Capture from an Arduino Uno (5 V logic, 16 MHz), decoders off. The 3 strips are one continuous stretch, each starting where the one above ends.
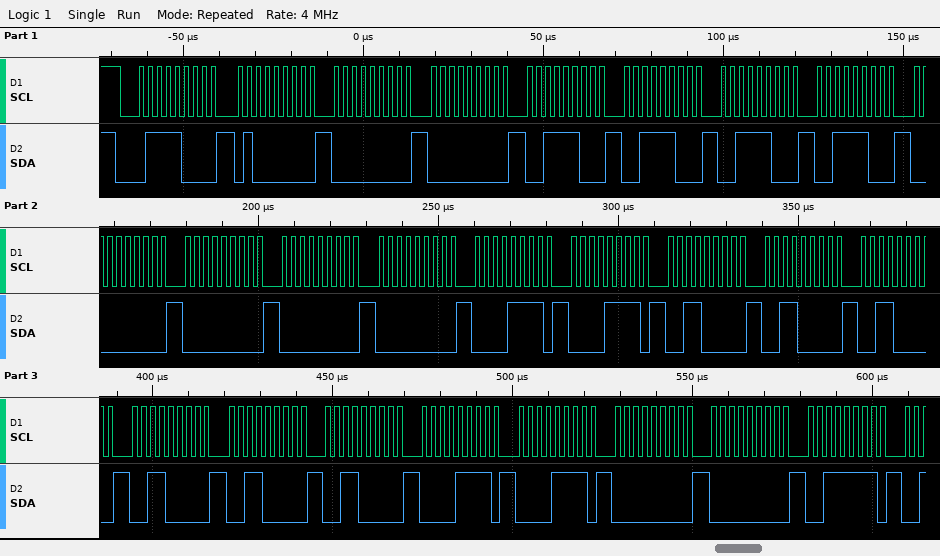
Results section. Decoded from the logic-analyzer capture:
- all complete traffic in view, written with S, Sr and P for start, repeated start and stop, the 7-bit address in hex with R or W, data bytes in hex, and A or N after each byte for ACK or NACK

S 3CW A 40 A 00 A 00 A 3C A 3C A 3C A 3C A 00 A 00 A 00 A 00 A 0F A 0F A 30 A 30 A 30 A 30 A 30 A 30 A 0F A 0F A 00 A 00 A 3F A
